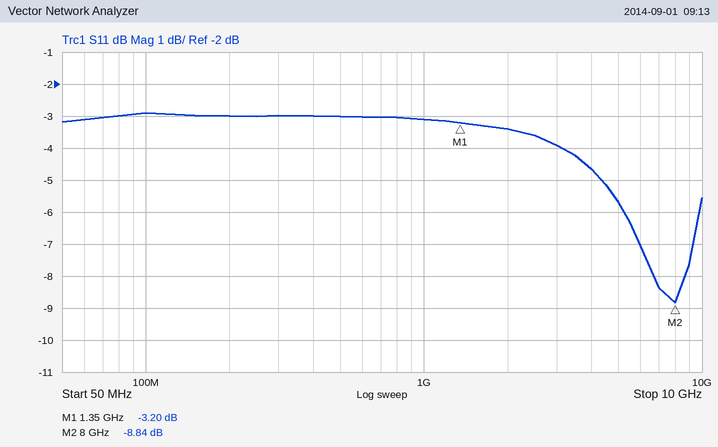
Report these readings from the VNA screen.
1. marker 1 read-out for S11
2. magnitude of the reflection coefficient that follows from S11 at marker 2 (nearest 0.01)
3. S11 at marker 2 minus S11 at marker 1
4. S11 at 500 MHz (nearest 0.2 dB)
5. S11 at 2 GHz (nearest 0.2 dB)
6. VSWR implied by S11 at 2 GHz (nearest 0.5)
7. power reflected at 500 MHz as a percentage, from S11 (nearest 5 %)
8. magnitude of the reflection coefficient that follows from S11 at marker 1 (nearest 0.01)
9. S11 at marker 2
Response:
-3.20 dB
0.36
-5.64 dB
-3.0 dB
-3.4 dB
5.0
50 %
0.69
-8.84 dB
